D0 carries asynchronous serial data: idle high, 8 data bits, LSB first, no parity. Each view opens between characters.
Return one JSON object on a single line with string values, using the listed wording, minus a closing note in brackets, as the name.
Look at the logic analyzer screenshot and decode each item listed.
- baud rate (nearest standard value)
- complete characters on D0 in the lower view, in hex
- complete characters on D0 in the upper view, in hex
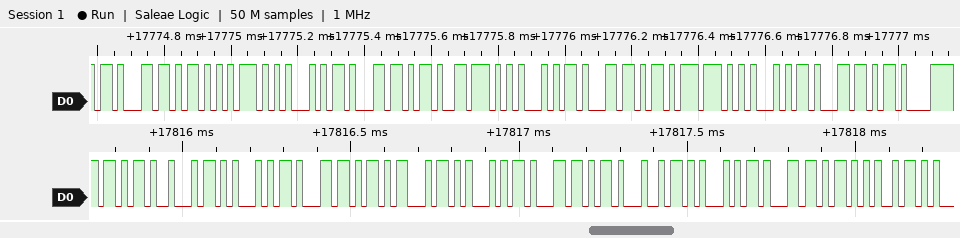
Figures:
{"baud rate": "57600 baud", "complete characters on D0 in the lower view, in hex": "6B, A2, 45, 8B, 6B, A3, 45, 8B, 6B, A4, 45, 8B, 6B, A5", "complete characters on D0 in the upper view, in hex": "8B, 6B, 75, 45, 8B, 6B, 76, 45, 8B, 6B, 77, 45, 8B, 6B"}
